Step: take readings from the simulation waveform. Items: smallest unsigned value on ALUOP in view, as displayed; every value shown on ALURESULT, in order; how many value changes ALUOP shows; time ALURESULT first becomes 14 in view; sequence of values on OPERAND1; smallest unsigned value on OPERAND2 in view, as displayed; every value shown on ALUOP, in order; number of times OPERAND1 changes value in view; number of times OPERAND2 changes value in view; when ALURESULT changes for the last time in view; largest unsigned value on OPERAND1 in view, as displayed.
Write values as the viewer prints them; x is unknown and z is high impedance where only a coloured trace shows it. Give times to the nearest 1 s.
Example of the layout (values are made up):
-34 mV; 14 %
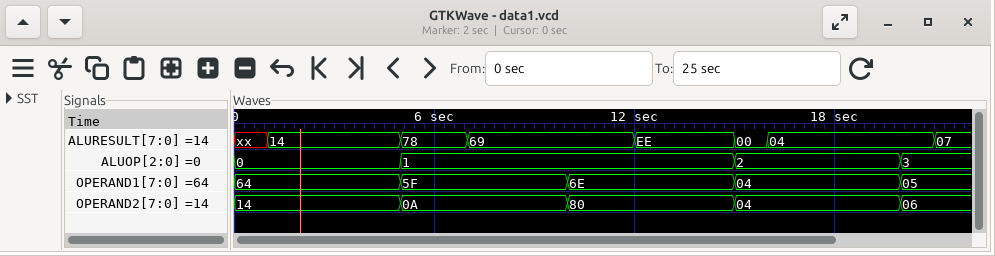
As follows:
0; xx, 14, 78, 69, EE, 00, 04, 07; 3; 1 s; 64, 5F, 6E, 04, 05; 04; 0, 1, 2, 3; 4; 4; 21 s; 6E
